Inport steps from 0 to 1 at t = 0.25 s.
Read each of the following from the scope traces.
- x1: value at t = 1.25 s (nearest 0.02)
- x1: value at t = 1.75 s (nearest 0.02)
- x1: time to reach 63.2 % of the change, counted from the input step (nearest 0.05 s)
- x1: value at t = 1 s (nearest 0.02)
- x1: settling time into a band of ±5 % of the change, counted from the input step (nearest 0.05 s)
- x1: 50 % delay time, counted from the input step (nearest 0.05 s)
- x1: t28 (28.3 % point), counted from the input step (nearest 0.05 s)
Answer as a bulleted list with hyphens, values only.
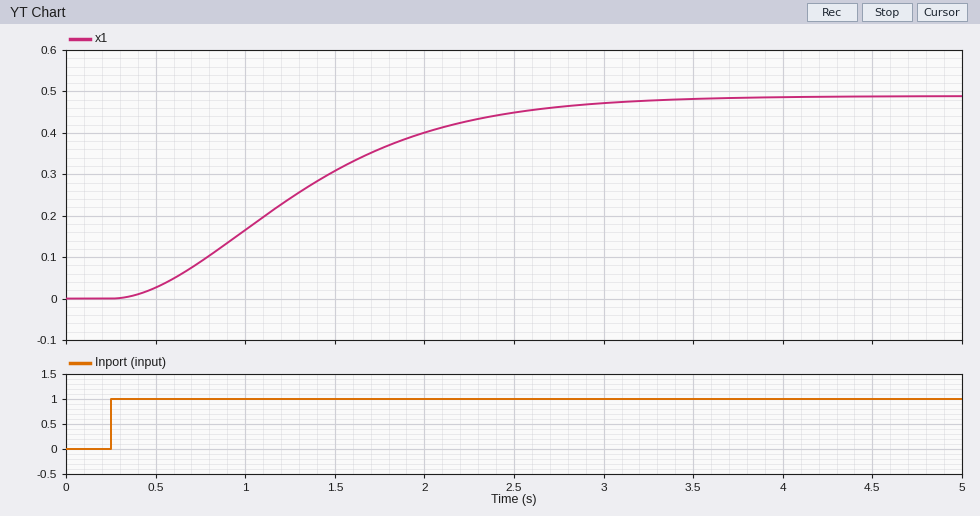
- 0.24
- 0.36
- 1.25 s
- 0.16
- 2.55 s
- 1.00 s
- 0.65 s
